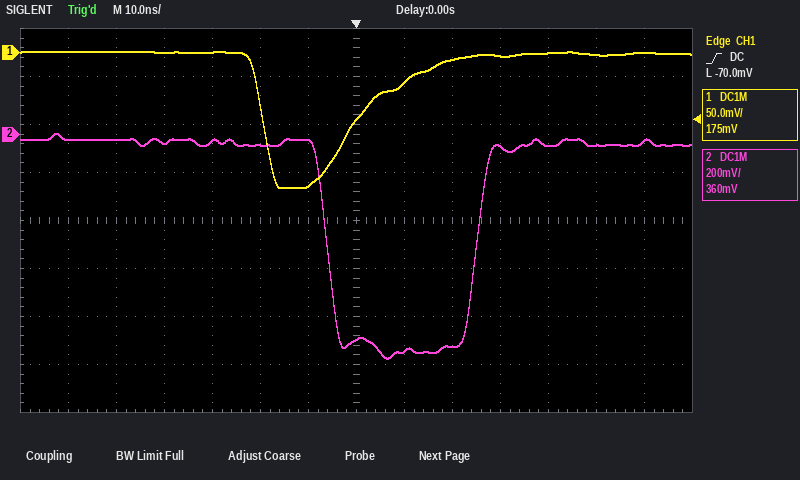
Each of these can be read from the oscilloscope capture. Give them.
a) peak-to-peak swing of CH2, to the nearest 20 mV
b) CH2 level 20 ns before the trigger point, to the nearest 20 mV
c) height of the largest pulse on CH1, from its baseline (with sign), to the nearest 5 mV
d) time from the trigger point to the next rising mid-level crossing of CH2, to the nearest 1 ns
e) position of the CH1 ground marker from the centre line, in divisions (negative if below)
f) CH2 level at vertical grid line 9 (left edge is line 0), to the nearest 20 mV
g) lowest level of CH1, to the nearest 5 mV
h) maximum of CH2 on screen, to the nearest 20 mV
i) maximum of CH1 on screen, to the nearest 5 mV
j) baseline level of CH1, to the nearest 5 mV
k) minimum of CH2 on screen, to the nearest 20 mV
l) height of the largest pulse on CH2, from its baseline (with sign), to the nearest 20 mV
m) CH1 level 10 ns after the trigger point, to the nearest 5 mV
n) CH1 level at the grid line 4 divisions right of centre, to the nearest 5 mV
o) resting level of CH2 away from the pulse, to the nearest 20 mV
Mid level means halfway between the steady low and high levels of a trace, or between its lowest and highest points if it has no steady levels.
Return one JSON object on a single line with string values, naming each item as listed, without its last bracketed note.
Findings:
{"peak-to-peak swing of CH2, to the nearest 20 mV": "940 mV", "CH2 level 20 ns before the trigger point, to the nearest 20 mV": "-40 mV", "height of the largest pulse on CH1, from its baseline (with sign), to the nearest 5 mV": "-140 mV", "time from the trigger point to the next rising mid-level crossing of CH2, to the nearest 1 ns": "25 ns", "position of the CH1 ground marker from the centre line, in divisions": "+3.5 div", "CH2 level at vertical grid line 9 (left edge is line 0), to the nearest 20 mV": "-880 mV", "lowest level of CH1, to the nearest 5 mV": "-140 mV", "maximum of CH2 on screen, to the nearest 20 mV": "0 mV", "maximum of CH1 on screen, to the nearest 5 mV": "0 mV", "baseline level of CH1, to the nearest 5 mV": "0 mV", "minimum of CH2 on screen, to the nearest 20 mV": "-940 mV", "height of the largest pulse on CH2, from its baseline (with sign), to the nearest 20 mV": "-900 mV", "CH1 level 10 ns after the trigger point, to the nearest 5 mV": "-30 mV", "CH1 level at the grid line 4 divisions right of centre, to the nearest 5 mV": "0 mV", "resting level of CH2 away from the pulse, to the nearest 20 mV": "-40 mV"}
